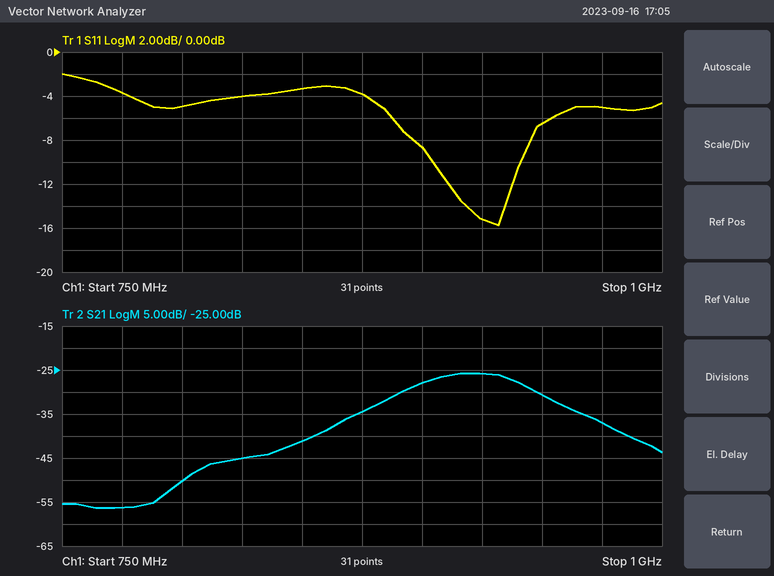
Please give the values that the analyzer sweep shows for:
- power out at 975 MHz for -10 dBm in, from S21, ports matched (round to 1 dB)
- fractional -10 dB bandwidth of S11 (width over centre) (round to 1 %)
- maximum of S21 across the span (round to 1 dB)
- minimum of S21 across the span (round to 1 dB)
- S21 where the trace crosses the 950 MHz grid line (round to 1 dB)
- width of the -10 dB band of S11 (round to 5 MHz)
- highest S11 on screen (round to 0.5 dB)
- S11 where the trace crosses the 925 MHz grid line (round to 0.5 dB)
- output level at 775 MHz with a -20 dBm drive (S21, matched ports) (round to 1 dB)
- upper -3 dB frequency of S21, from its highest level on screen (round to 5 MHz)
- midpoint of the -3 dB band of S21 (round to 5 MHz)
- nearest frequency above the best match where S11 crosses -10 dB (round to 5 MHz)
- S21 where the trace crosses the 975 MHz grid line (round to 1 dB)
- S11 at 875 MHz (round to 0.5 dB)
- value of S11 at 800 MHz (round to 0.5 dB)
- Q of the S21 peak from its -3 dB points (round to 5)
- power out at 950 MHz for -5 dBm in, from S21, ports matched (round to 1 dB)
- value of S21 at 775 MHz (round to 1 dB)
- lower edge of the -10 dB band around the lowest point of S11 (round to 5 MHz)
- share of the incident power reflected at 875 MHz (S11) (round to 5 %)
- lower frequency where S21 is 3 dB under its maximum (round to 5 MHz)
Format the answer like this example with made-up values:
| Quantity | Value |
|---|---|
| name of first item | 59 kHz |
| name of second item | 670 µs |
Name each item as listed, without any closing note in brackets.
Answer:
| Quantity | Value |
|---|---|
| power out at 975 MHz for -10 dBm in, from S21, ports matched | -47 dBm |
| fractional -10 dB bandwidth of S11 (width over centre) | 4 % |
| maximum of S21 across the span | -26 dB |
| minimum of S21 across the span | -56 dB |
| S21 where the trace crosses the 950 MHz grid line | -31 dB |
| width of the -10 dB band of S11 | 35 MHz |
| highest S11 on screen | -2.0 dB |
| S11 where the trace crosses the 925 MHz grid line | -15.0 dB |
| output level at 775 MHz with a -20 dBm drive (S21, matched ports) | -76 dBm |
| upper -3 dB frequency of S21, from its highest level on screen | 945 MHz |
| midpoint of the -3 dB band of S21 | 920 MHz |
| nearest frequency above the best match where S11 crosses -10 dB | 940 MHz |
| S21 where the trace crosses the 975 MHz grid line | -37 dB |
| S11 at 875 MHz | -4.0 dB |
| value of S11 at 800 MHz | -5.0 dB |
| Q of the S21 peak from its -3 dB points | 20 |
| power out at 950 MHz for -5 dBm in, from S21, ports matched | -36 dBm |
| value of S21 at 775 MHz | -56 dB |
| lower edge of the -10 dB band around the lowest point of S11 | 905 MHz |
| share of the incident power reflected at 875 MHz (S11) | 40 % |
| lower frequency where S21 is 3 dB under its maximum | 895 MHz |
